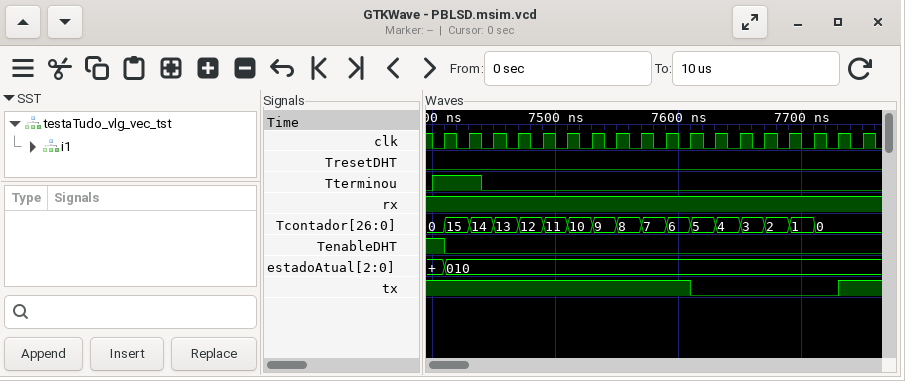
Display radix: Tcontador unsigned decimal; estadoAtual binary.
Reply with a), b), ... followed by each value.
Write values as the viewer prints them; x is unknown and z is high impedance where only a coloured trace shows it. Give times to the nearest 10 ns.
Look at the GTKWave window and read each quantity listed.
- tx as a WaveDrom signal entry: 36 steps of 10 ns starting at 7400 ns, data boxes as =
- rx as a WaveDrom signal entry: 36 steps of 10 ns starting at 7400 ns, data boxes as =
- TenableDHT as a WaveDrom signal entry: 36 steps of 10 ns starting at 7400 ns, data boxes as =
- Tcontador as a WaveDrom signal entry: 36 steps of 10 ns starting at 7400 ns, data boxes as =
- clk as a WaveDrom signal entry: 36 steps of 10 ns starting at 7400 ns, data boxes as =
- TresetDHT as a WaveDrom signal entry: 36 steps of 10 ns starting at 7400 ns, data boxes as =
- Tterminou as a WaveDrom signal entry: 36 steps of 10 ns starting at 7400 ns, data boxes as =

a) {name: 'tx', wave: '1....................0...........1..'}
b) {name: 'rx', wave: '1...................................'}
c) {name: 'TenableDHT', wave: '10..................................'}
d) {name: 'Tcontador', wave: '==.=.=.=.=.=.=.=.=.=.=.=.=.=.=.=....', data: '0 15 14 13 12 11 10 9 8 7 6 5 4 3 2 1 0'}
e) {name: 'clk', wave: '010101010101010101010101010101010101'}
f) {name: 'TresetDHT', wave: '0...................................'}
g) {name: 'Tterminou', wave: '1...0...............................'}
